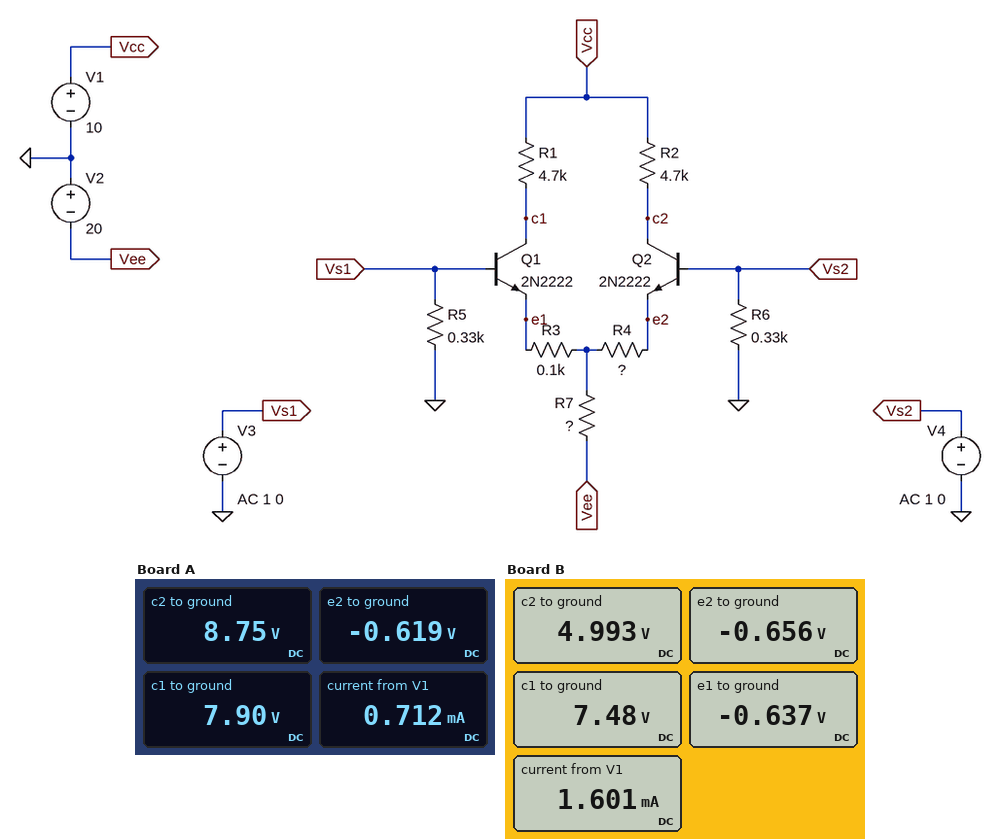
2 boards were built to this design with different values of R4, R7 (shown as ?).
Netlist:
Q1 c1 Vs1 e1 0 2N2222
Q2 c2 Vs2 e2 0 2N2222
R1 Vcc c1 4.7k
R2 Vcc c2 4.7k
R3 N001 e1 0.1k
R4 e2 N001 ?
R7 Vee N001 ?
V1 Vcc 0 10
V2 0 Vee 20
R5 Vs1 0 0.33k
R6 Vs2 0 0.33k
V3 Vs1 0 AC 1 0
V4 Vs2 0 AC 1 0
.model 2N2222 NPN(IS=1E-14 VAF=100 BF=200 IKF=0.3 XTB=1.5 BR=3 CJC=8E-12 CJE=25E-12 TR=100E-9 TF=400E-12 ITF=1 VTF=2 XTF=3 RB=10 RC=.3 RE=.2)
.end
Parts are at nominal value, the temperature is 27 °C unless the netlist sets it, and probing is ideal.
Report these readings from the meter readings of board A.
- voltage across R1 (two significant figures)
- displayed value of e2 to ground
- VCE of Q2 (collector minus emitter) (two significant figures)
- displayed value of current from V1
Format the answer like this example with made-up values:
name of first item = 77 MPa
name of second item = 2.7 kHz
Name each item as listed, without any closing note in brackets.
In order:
voltage across R1 = 2.1 V
displayed value of e2 to ground = -0.619 V
VCE of Q2 (collector minus emitter) = 9.4 V
displayed value of current from V1 = 0.712 mA
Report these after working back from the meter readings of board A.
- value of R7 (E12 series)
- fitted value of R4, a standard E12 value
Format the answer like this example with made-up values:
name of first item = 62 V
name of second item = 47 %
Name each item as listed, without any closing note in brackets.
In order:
value of R7 = 27 kΩ
fitted value of R4, a standard E12 value = 220 Ω
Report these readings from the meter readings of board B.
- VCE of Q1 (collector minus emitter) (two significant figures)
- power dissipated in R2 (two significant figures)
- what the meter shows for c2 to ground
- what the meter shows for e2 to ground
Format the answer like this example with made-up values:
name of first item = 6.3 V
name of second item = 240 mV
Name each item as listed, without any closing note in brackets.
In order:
VCE of Q1 (collector minus emitter) = 8.1 V
power dissipated in R2 = 5.3 mW
what the meter shows for c2 to ground = 4.993 V
what the meter shows for e2 to ground = -0.656 V
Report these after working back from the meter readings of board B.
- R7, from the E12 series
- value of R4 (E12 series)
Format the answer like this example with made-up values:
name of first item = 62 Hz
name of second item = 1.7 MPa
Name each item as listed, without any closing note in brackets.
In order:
R7, from the E12 series = 12 kΩ
value of R4 = 33 Ω
